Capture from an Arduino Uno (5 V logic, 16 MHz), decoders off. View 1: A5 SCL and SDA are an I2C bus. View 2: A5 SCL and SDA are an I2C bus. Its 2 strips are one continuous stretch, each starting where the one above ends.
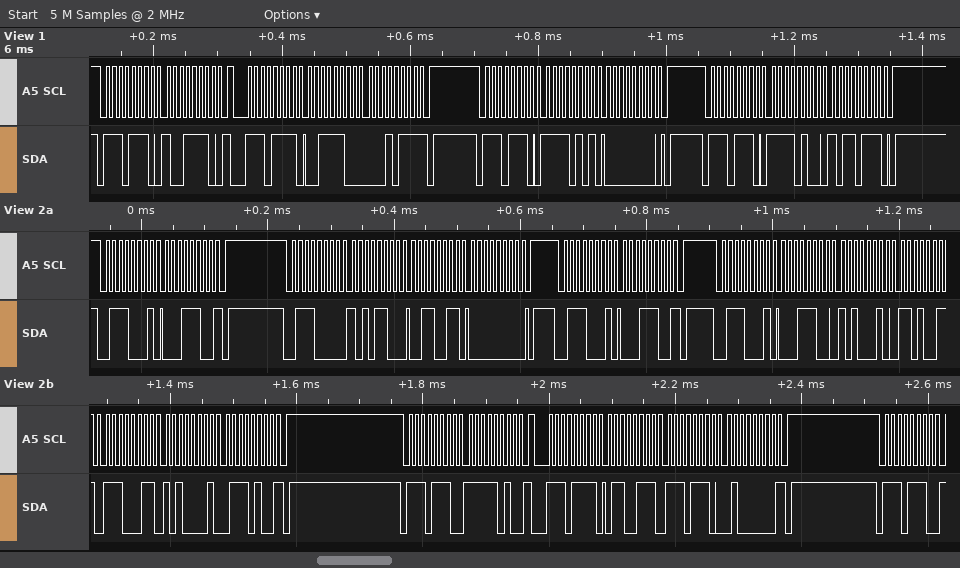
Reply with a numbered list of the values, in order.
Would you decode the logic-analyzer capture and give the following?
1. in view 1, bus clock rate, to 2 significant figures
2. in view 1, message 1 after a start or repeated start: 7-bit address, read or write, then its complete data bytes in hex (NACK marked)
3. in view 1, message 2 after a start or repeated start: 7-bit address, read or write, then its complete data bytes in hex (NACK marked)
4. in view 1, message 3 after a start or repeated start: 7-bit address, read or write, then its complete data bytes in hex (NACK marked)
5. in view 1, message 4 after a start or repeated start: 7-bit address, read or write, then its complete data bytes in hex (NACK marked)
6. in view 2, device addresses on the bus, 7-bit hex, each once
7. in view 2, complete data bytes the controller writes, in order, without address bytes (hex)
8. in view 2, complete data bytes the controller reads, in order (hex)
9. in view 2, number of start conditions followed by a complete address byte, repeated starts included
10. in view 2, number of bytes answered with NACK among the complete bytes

1. 100 kHz
2. 0x77 write: 9E
3. 0x77 read: 3C 17 NACK
4. 0x77 write: F5 00
5. 0x77 write: F4 B7
6. 0x38 0x77
7. AC 33 00 FA
8. 1C 1C 1C A2 D3 E3 A1 74 67 EE 40
9. 7
10. 4
